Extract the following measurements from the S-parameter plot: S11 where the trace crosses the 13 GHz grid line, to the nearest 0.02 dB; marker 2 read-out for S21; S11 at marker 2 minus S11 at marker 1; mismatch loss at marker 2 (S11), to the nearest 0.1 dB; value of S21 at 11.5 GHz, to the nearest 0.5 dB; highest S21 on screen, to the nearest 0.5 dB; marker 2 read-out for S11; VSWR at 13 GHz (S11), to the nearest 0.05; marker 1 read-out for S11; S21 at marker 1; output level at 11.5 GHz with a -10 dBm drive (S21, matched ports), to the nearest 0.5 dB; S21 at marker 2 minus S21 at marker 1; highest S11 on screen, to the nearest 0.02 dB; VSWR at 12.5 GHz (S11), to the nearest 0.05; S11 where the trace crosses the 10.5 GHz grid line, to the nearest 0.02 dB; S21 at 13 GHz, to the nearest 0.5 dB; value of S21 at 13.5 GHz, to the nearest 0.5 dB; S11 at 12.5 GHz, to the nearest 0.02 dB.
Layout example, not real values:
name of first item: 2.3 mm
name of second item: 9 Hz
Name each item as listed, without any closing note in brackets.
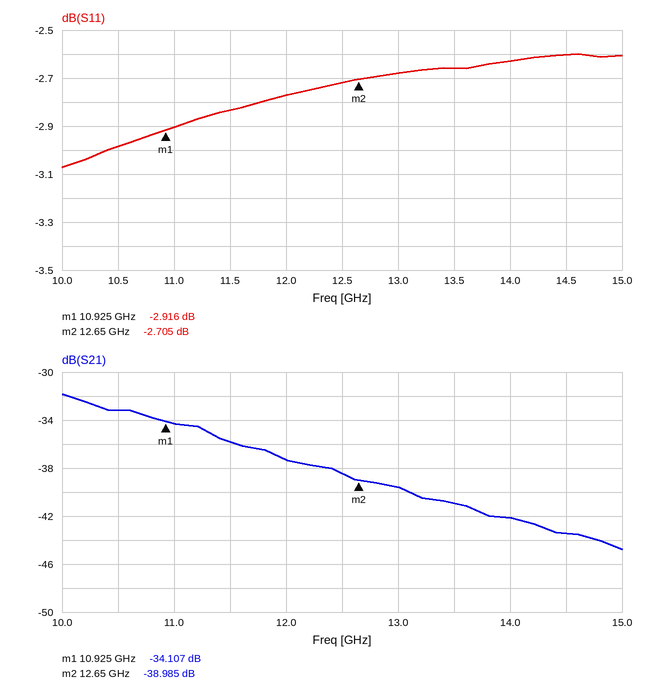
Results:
S11 where the trace crosses the 13 GHz grid line, to the nearest 0.02 dB: -2.68 dB
marker 2 read-out for S21: -38.985 dB
S11 at marker 2 minus S11 at marker 1: 0.211 dB
mismatch loss at marker 2 (S11), to the nearest 0.1 dB: 3.3 dB
value of S21 at 11.5 GHz, to the nearest 0.5 dB: -36.0 dB
highest S21 on screen, to the nearest 0.5 dB: -32.0 dB
marker 2 read-out for S11: -2.705 dB
VSWR at 13 GHz (S11), to the nearest 0.05: 6.55
marker 1 read-out for S11: -2.916 dB
S21 at marker 1: -34.107 dB
output level at 11.5 GHz with a -10 dBm drive (S21, matched ports), to the nearest 0.5 dB: -46.0 dBm
S21 at marker 2 minus S21 at marker 1: -4.878 dB
highest S11 on screen, to the nearest 0.02 dB: -2.60 dB
VSWR at 12.5 GHz (S11), to the nearest 0.05: 6.45
S11 where the trace crosses the 10.5 GHz grid line, to the nearest 0.02 dB: -2.98 dB
S21 at 13 GHz, to the nearest 0.5 dB: -39.5 dB
value of S21 at 13.5 GHz, to the nearest 0.5 dB: -41.0 dB
S11 at 12.5 GHz, to the nearest 0.02 dB: -2.72 dB
